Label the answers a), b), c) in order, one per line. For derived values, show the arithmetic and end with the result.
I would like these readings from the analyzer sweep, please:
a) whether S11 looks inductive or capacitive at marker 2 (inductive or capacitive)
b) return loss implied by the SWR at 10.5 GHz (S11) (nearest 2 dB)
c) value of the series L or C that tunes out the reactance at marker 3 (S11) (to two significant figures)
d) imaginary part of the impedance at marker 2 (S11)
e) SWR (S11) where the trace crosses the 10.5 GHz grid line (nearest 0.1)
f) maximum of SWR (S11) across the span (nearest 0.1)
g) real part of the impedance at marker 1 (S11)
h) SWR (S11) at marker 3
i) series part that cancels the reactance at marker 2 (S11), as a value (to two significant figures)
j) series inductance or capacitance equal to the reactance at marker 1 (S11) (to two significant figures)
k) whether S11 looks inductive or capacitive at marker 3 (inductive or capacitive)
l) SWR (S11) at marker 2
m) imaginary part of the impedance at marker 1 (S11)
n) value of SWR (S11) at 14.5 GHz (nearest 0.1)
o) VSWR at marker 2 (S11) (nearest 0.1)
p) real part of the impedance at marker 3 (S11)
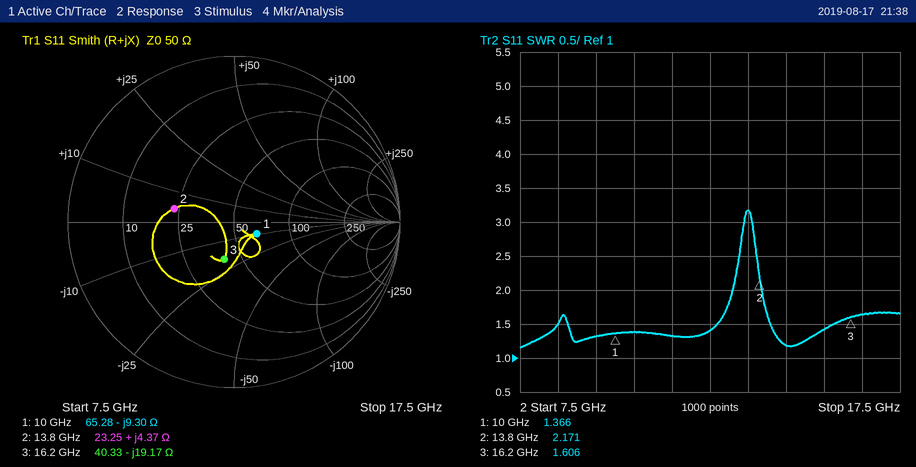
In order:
a) inductive
b) −20 log10((1.4 − 1)/(1.4 + 1)) ≈ 16 dB
c) L = 19.17 Ω/(2π × 16.2 GHz) ≈ 188 pH, so 190 pH to two significant figures
d) +4.37 Ω
e) 1.4
f) 3.2
g) 65.28 Ω
h) 1.606
i) C = 1/(2π × 13.8 GHz × 4.37 Ω) ≈ 2.6 pF
j) C = 1/(2π × 10 GHz × 9.3 Ω) ≈ 1.7 pF
k) capacitive
l) 2.171
m) -9.30 Ω
n) 1.2
o) 2.2
p) 40.33 Ω
